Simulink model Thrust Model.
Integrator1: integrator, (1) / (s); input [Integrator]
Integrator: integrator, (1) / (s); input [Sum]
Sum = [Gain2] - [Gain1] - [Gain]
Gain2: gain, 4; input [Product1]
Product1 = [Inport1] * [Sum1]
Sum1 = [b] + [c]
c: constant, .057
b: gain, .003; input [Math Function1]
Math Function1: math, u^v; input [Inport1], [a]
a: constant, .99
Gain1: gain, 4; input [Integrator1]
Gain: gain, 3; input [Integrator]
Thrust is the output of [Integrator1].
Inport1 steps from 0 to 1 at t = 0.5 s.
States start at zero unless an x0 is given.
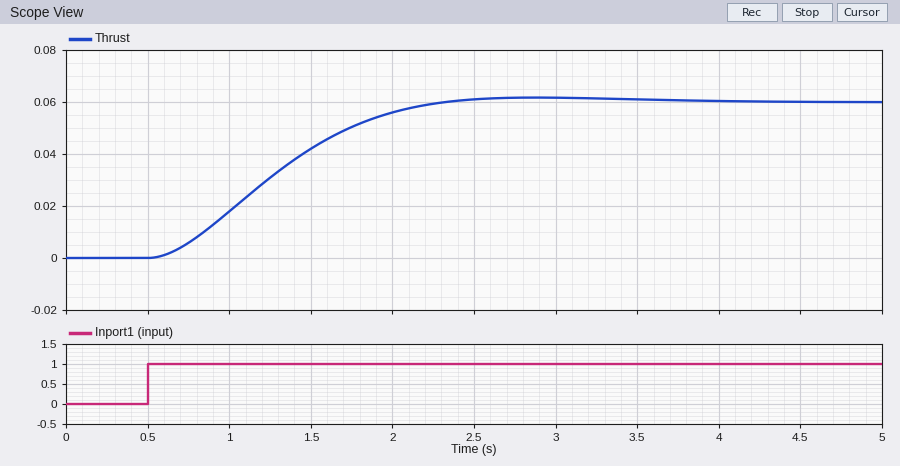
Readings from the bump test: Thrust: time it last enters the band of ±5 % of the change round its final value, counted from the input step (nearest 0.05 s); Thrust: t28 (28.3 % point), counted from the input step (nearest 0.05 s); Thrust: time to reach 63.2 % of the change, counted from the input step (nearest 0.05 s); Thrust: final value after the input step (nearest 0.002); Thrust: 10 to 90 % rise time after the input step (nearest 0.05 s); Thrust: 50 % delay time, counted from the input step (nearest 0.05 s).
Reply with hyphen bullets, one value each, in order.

- 1.55 s
- 0.50 s
- 0.90 s
- 0.060
- 1.15 s
- 0.75 s
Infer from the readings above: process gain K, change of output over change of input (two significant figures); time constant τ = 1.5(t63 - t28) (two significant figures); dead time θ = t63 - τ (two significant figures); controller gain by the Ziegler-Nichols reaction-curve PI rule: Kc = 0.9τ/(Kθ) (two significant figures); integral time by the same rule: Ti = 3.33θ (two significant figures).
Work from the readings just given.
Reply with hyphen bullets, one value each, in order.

- 0.060
- 0.60 s
- 0.30 s
- 30
- 1.00 s
